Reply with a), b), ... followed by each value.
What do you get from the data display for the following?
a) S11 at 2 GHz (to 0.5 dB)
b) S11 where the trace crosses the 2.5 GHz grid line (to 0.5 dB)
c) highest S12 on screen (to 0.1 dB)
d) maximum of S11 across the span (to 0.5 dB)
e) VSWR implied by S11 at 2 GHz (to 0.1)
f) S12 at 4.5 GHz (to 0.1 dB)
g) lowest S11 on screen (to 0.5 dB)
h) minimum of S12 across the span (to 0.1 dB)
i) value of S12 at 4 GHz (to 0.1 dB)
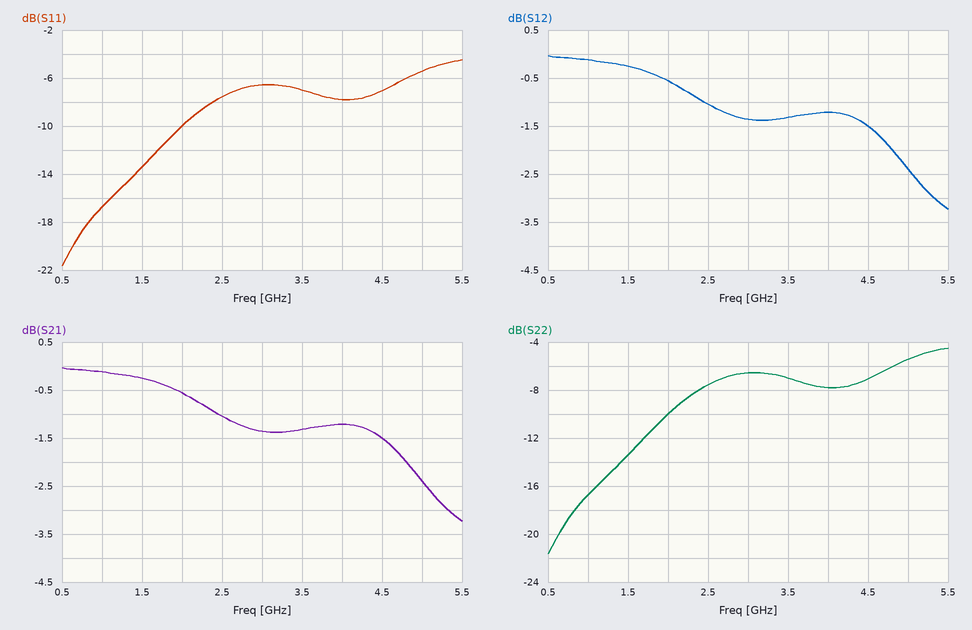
a) -10.0 dB
b) -7.5 dB
c) 0.0 dB
d) -4.5 dB
e) 1.9
f) -1.5 dB
g) -21.5 dB
h) -3.2 dB
i) -1.2 dB
